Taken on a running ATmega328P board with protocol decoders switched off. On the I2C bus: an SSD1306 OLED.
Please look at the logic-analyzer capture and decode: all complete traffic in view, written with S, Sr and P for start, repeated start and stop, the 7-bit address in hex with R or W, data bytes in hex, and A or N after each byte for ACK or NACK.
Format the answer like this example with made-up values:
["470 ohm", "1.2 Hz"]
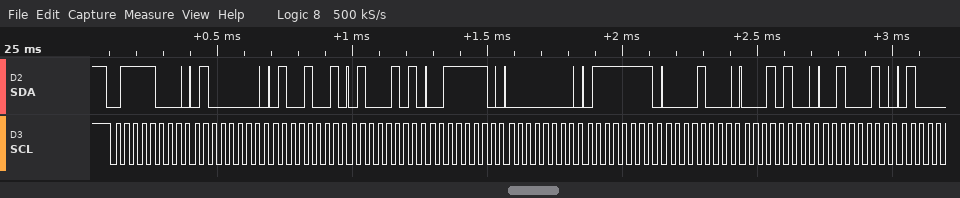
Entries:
["S 3CW A 40 A 49 A 45 A 3E A 00 A 7F A 08 A 14 A 22 A"]
